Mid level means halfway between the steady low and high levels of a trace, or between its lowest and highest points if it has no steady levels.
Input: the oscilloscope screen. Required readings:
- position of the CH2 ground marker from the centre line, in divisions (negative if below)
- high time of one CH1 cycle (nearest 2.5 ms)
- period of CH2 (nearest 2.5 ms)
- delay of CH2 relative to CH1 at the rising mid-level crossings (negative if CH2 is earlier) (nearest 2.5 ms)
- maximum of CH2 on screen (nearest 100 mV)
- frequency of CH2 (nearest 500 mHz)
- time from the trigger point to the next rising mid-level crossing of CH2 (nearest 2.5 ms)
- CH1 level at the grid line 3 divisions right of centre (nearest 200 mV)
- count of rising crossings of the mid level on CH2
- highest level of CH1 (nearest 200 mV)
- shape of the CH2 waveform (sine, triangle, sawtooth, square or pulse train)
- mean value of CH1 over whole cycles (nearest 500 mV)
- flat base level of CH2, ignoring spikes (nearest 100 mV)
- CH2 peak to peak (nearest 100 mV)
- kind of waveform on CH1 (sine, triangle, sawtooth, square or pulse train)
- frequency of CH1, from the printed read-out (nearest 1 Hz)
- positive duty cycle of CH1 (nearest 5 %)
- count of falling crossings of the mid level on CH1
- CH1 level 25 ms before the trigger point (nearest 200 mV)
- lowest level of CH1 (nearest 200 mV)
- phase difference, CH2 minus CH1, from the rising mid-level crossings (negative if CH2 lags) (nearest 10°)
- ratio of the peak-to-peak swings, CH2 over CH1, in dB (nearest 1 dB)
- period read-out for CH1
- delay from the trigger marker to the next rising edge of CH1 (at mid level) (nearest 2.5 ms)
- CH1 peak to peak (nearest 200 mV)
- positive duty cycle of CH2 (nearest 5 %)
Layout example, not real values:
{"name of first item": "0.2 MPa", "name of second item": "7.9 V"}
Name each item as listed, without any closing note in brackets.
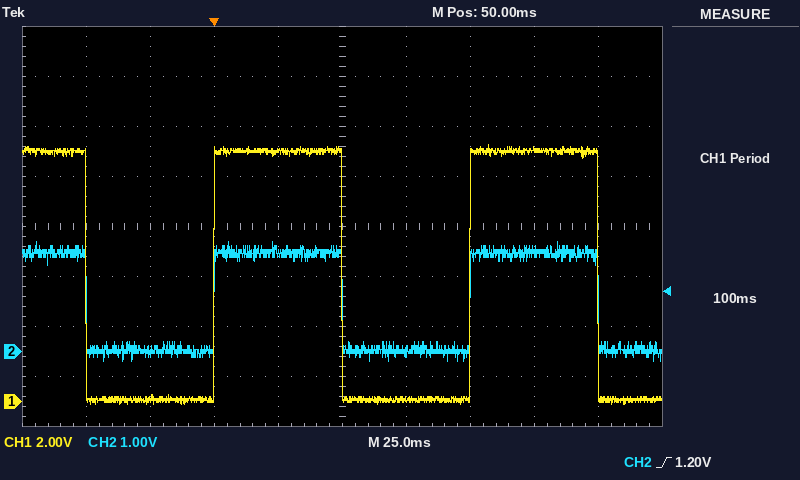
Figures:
{"position of the CH2 ground marker from the centre line, in divisions": "-2.5 div", "high time of one CH1 cycle": "50.0 ms", "period of CH2": "100.0 ms", "delay of CH2 relative to CH1 at the rising mid-level crossings (negative if CH2 is earlier)": "0.0 ms", "maximum of CH2 on screen": "2.2 V", "frequency of CH2": "10.0 Hz", "time from the trigger point to the next rising mid-level crossing of CH2": "100.0 ms", "CH1 level at the grid line 3 divisions right of centre": "10.0 V", "count of rising crossings of the mid level on CH2": "2", "highest level of CH1": "10.2 V", "shape of the CH2 waveform": "square", "mean value of CH1 over whole cycles": "5.0 V", "flat base level of CH2, ignoring spikes": "0.0 V", "CH2 peak to peak": "2.4 V", "kind of waveform on CH1": "square", "frequency of CH1, from the printed read-out": "10 Hz", "positive duty cycle of CH1": "50 %", "count of falling crossings of the mid level on CH1": "3", "CH1 level 25 ms before the trigger point": "200 mV", "lowest level of CH1": "-200 mV", "phase difference, CH2 minus CH1, from the rising mid-level crossings (negative if CH2 lags)": "0°", "ratio of the peak-to-peak swings, CH2 over CH1, in dB": "-13 dB", "period read-out for CH1": "100 ms", "delay from the trigger marker to the next rising edge of CH1 (at mid level)": "100.0 ms", "CH1 peak to peak": "10.4 V", "positive duty cycle of CH2": "50 %"}
